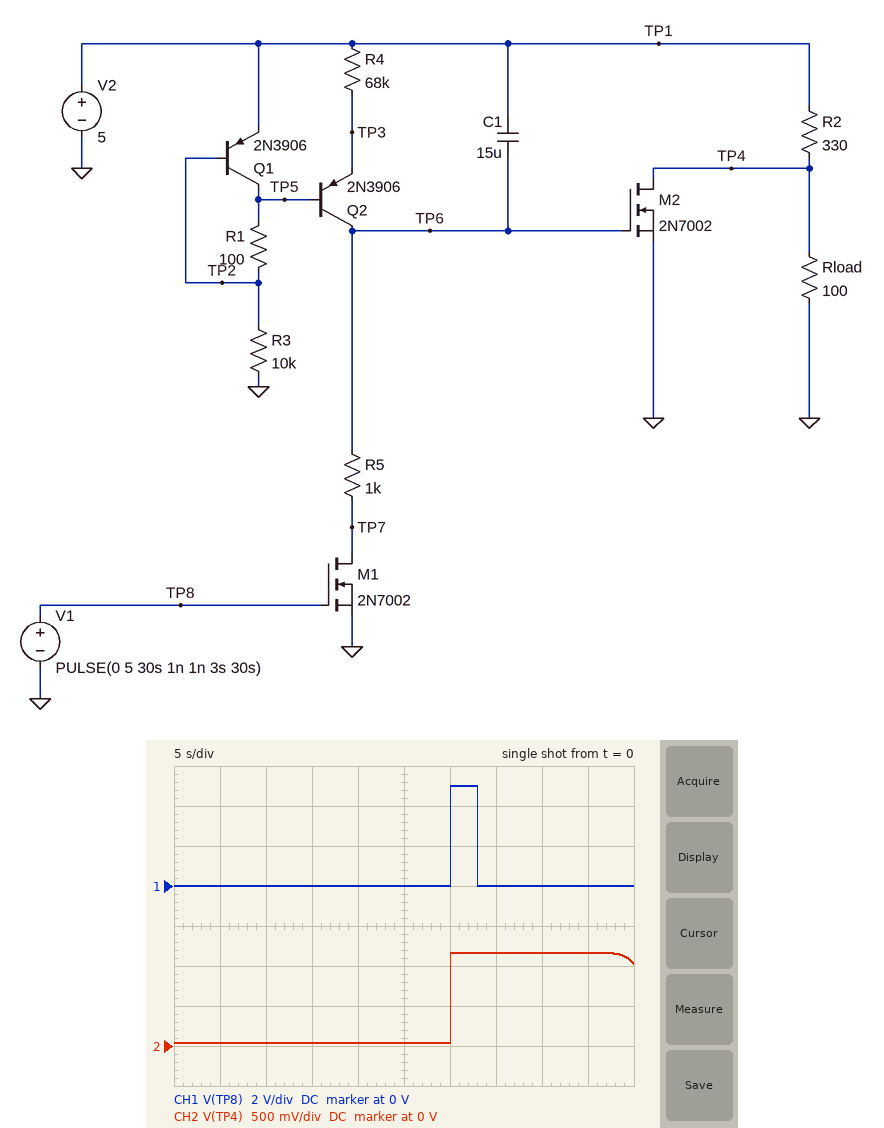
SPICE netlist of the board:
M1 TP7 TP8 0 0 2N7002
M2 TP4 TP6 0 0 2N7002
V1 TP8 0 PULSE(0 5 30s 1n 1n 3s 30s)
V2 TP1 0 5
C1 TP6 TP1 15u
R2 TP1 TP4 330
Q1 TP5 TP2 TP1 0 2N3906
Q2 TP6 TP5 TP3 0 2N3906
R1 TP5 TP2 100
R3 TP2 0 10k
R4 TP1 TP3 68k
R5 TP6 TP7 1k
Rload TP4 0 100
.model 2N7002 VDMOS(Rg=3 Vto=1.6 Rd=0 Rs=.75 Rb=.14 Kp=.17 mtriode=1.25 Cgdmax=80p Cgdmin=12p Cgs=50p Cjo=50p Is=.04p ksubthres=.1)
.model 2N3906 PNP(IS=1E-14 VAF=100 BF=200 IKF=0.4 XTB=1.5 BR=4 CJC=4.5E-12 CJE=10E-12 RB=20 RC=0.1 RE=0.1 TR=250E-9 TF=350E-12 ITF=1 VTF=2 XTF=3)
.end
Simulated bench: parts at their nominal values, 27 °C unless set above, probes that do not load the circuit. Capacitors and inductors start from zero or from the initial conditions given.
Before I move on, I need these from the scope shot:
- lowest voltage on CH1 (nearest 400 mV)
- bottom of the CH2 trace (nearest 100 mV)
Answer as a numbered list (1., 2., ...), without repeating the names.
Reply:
1. 0 V
2. 0 V
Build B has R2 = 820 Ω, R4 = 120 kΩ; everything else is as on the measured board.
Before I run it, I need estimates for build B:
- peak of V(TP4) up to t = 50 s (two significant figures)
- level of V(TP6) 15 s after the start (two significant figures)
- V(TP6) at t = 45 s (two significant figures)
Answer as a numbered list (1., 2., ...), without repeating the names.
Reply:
1. 540 mV
2. 4.9 V
3. 770 mV
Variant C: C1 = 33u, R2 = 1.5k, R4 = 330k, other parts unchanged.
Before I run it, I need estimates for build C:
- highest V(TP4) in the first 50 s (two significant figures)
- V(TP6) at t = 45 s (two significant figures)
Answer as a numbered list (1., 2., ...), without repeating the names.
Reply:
1. 310 mV
2. 150 mV
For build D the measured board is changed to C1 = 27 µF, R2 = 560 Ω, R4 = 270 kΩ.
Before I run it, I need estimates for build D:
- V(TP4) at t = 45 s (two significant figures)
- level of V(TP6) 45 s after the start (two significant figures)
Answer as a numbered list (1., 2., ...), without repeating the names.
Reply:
1. 760 mV
2. 220 mV
